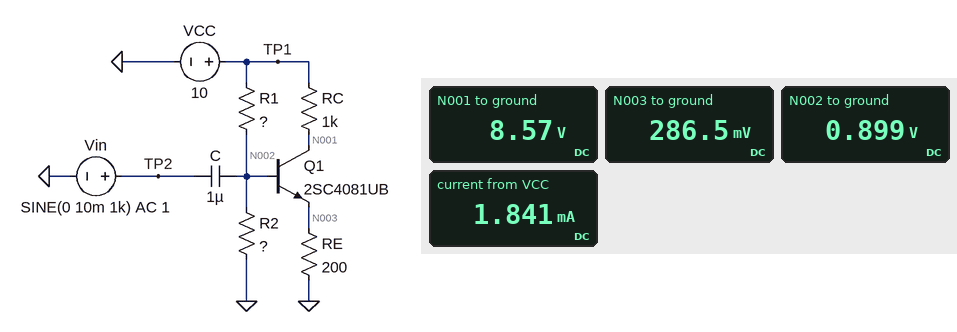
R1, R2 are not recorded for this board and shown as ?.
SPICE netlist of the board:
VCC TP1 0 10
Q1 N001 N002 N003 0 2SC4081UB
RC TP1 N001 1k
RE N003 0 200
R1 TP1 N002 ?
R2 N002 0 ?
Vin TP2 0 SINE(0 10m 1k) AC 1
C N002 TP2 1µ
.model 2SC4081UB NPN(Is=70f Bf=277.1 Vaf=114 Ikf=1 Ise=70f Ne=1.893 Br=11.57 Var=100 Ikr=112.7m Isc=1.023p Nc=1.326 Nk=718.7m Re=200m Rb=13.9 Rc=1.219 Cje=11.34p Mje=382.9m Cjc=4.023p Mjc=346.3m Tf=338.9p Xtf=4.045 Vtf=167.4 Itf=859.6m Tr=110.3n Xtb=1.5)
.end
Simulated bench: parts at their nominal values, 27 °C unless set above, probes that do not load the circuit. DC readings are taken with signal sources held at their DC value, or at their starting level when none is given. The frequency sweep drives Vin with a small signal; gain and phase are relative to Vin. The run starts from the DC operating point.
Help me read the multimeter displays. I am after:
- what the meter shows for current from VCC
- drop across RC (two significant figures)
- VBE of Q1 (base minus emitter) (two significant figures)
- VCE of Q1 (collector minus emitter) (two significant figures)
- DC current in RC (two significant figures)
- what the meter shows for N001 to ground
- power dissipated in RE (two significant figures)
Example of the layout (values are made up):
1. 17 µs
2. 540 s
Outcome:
1. 1.841 mA
2. 1.4 V
3. 610 mV
4. 8.3 V
5. 1.4 mA
6. 8.57 V
7. 410 µW
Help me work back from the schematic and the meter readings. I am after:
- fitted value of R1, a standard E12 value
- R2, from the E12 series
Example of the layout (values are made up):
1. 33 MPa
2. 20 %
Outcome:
1. 22 kΩ
2. 2.2 kΩ
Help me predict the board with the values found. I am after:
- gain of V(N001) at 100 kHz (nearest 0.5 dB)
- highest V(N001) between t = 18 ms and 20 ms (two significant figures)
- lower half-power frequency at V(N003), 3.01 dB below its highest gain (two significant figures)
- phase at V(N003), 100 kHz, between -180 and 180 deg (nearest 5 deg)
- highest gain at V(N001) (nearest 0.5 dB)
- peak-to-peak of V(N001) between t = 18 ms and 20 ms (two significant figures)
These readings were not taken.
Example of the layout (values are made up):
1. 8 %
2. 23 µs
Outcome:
1. 13.0 dB
2. 8.6 V
3. 82 Hz
4. 0 deg
5. 13.0 dB
6. 91 mV
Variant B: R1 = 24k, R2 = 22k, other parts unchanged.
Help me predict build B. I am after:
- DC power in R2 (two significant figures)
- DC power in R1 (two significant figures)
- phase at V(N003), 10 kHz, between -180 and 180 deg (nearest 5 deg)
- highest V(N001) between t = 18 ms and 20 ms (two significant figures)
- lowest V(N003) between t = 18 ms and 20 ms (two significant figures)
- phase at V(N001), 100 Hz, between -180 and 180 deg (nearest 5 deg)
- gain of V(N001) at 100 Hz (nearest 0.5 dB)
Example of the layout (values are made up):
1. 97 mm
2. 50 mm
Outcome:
1. 250 µW
2. 2.4 mW
3. 5 deg
4. 1.8 V
5. 1.7 V
6. 80 deg
7. -29.0 dB
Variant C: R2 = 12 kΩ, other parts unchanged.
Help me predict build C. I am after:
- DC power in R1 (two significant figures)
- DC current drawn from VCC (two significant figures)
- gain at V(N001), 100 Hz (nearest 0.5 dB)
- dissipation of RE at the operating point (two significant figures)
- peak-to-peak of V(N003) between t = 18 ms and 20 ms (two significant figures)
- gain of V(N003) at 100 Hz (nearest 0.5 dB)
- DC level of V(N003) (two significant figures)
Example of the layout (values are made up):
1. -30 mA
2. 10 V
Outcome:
1. 2.7 mW
2. 8.6 mA
3. -51.5 dB
4. 14 mW
5. 14 mV
6. -18.5 dB
7. 1.7 V
